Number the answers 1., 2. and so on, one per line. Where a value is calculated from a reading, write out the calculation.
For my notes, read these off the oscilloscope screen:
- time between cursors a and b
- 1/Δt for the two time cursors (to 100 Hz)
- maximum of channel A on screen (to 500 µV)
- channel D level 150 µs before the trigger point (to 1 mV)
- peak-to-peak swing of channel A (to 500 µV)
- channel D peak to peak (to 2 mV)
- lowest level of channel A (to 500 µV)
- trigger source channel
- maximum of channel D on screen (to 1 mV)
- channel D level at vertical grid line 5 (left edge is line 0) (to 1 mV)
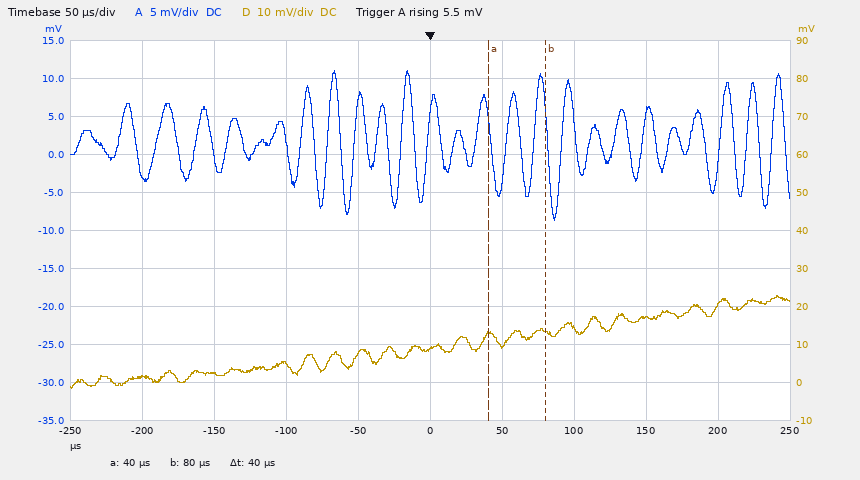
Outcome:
1. 40 µs
2. 1 / 40 µs ≈ 25.0 kHz
3. 11.0 mV
4. 2 mV
5. 11.0 mV − (-8.5 mV) = 19.5 mV
6. 24 mV
7. -8.5 mV
8. channel A
9. 23 mV
10. 9 mV
